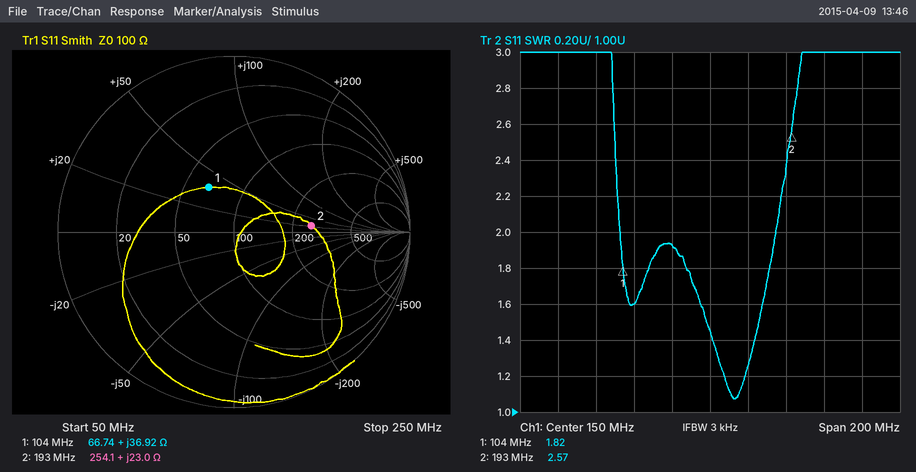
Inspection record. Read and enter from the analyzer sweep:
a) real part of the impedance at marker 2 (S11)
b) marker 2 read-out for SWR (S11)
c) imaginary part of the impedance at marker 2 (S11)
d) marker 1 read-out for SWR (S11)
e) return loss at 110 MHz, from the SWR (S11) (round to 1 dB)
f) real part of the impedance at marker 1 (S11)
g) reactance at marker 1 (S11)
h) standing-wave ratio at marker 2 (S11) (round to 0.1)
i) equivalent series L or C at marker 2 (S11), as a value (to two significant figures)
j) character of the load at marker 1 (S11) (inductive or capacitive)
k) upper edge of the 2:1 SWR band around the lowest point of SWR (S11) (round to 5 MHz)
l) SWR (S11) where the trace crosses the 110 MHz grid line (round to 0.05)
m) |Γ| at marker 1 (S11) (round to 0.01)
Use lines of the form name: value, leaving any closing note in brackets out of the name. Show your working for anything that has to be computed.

real part of the impedance at marker 2: 254.1 Ω
marker 2 read-out for SWR: 2.57
imaginary part of the impedance at marker 2: +23.0 Ω
marker 1 read-out for SWR: 1.82
return loss at 110 MHz, from the SWR (S11): −20 log10((1.6 − 1)/(1.6 + 1)) ≈ 13 dB
real part of the impedance at marker 1: 66.74 Ω
reactance at marker 1: +36.92 Ω
standing-wave ratio at marker 2 (S11): 2.6
equivalent series L or C at marker 2 (S11), as a value: L = 23 Ω/(2π × 193 MHz) ≈ 19 nH
character of the load at marker 1 (S11): inductive
upper edge of the 2:1 SWR band around the lowest point of SWR (S11): 185 MHz
SWR (S11) where the trace crosses the 110 MHz grid line: 1.60
|Γ| at marker 1 (S11): 0.29
